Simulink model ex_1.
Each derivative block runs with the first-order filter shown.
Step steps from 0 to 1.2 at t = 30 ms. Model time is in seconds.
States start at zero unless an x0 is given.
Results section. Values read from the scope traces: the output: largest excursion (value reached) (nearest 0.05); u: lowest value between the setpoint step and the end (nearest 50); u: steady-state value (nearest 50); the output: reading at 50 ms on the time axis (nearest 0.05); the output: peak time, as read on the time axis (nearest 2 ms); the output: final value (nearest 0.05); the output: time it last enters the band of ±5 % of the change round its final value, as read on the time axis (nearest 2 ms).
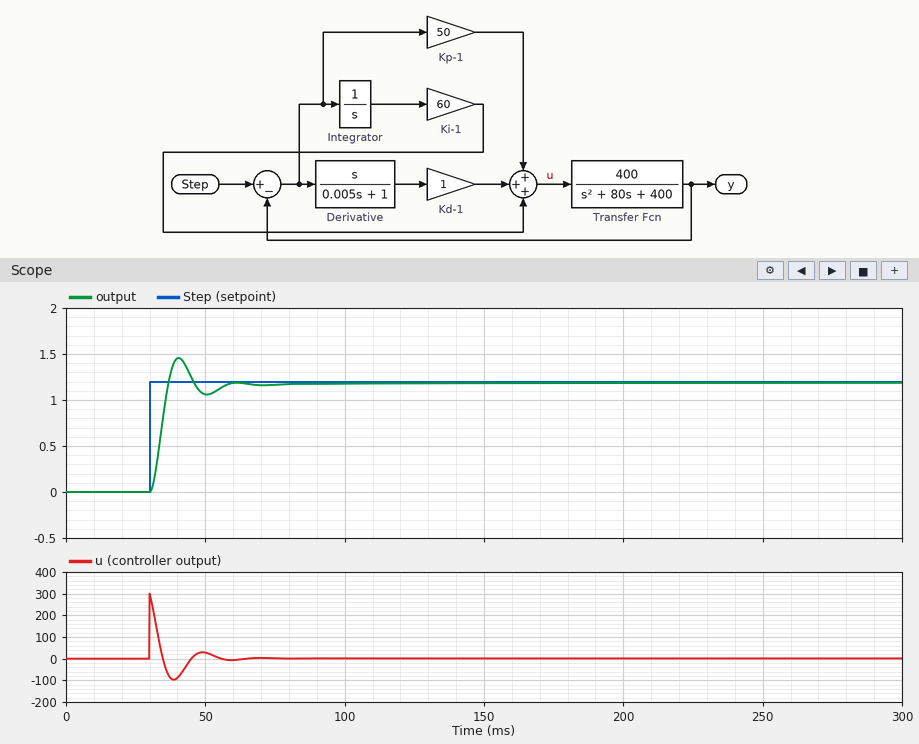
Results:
1.45
-100
0
1.05
40 ms
1.20
56 ms
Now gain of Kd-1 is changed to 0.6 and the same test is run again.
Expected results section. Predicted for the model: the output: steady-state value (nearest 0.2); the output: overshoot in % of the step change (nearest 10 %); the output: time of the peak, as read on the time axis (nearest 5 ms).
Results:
1.2
20 %
45 ms
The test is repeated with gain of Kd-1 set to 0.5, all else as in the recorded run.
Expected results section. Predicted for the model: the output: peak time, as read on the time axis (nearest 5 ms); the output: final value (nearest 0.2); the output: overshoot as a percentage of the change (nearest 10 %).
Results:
45 ms
1.2
20 %
